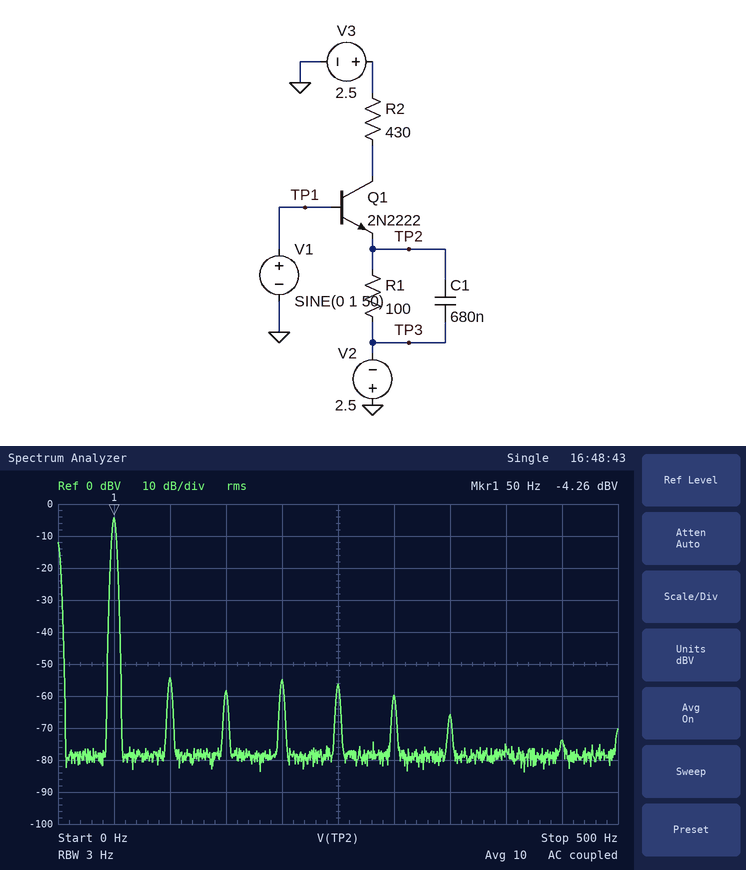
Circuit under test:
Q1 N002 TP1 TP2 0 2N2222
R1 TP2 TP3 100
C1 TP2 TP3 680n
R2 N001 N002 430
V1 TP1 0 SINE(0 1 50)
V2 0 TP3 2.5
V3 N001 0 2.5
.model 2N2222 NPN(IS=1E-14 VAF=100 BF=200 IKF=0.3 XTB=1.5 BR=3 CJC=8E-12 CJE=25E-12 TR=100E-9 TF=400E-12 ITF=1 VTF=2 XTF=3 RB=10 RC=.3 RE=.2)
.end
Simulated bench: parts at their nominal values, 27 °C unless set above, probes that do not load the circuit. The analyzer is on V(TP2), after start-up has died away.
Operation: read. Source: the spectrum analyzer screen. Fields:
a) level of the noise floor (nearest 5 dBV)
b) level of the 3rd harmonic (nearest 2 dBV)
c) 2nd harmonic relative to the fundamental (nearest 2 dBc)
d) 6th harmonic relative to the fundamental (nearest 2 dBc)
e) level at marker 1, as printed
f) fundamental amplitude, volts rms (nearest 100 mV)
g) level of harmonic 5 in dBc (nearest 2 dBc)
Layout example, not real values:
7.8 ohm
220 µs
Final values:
-80 dBV
-58 dBV
-50 dBc
-56 dBc
-4.26 dBV
600 mV
-52 dBc
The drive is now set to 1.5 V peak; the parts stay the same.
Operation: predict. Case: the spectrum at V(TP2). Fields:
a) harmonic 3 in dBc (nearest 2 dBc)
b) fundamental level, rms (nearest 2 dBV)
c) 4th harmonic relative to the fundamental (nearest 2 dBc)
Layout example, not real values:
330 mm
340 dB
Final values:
-42 dBc
0 dBV
-50 dBc
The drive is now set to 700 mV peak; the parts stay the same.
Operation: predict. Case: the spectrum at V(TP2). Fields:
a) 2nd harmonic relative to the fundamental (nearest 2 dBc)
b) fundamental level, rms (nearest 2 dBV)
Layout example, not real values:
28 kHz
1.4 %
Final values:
-46 dBc
-8 dBV
